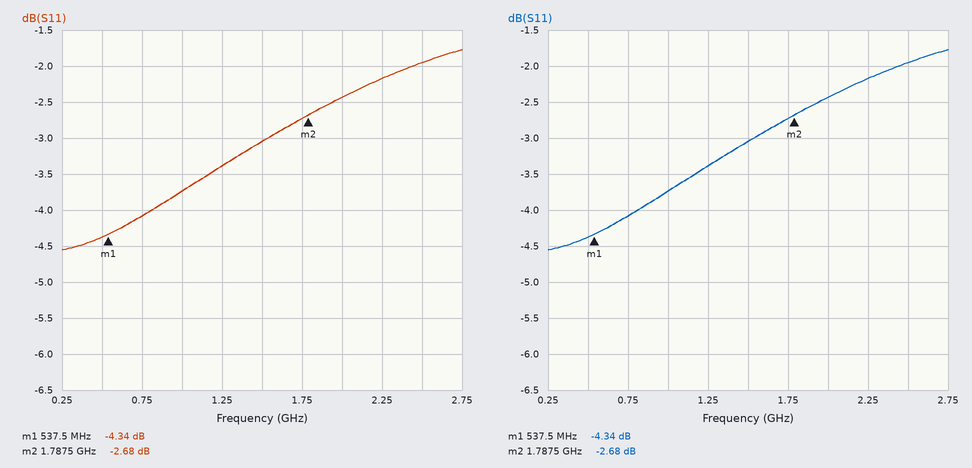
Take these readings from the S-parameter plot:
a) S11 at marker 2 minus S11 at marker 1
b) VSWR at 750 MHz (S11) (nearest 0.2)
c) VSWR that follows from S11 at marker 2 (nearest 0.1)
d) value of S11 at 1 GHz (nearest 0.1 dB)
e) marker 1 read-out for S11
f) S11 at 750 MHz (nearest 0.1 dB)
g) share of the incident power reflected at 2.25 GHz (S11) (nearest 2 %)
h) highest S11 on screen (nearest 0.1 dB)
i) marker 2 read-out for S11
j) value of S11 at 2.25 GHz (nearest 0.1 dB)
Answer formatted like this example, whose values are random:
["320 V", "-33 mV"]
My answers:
["1.66 dB", "4.4", "6.5", "-3.7 dB", "-4.34 dB", "-4.1 dB", "60 %", "-1.8 dB", "-2.68 dB", "-2.2 dB"]
